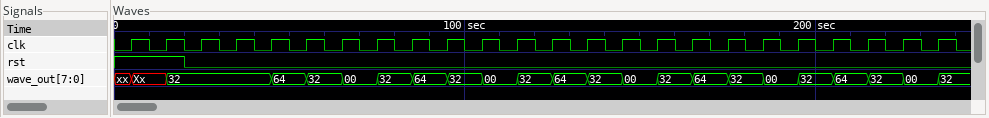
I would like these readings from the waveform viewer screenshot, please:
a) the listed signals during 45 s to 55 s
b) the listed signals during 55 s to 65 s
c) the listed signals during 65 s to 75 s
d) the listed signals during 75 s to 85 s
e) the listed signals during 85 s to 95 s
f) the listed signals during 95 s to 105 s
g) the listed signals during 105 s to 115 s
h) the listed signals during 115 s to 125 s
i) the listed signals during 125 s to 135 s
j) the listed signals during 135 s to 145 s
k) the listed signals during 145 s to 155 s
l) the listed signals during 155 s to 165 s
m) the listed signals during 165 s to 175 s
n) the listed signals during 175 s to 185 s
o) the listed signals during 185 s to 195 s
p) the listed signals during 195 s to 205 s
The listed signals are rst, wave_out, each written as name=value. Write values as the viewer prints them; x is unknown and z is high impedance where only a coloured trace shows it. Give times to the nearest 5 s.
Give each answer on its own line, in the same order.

rst=0, wave_out=64
rst=0, wave_out=32
rst=0, wave_out=00
rst=0, wave_out=32
rst=0, wave_out=64
rst=0, wave_out=32
rst=0, wave_out=00
rst=0, wave_out=32
rst=0, wave_out=64
rst=0, wave_out=32
rst=0, wave_out=00
rst=0, wave_out=32
rst=0, wave_out=64
rst=0, wave_out=32
rst=0, wave_out=00
rst=0, wave_out=32
